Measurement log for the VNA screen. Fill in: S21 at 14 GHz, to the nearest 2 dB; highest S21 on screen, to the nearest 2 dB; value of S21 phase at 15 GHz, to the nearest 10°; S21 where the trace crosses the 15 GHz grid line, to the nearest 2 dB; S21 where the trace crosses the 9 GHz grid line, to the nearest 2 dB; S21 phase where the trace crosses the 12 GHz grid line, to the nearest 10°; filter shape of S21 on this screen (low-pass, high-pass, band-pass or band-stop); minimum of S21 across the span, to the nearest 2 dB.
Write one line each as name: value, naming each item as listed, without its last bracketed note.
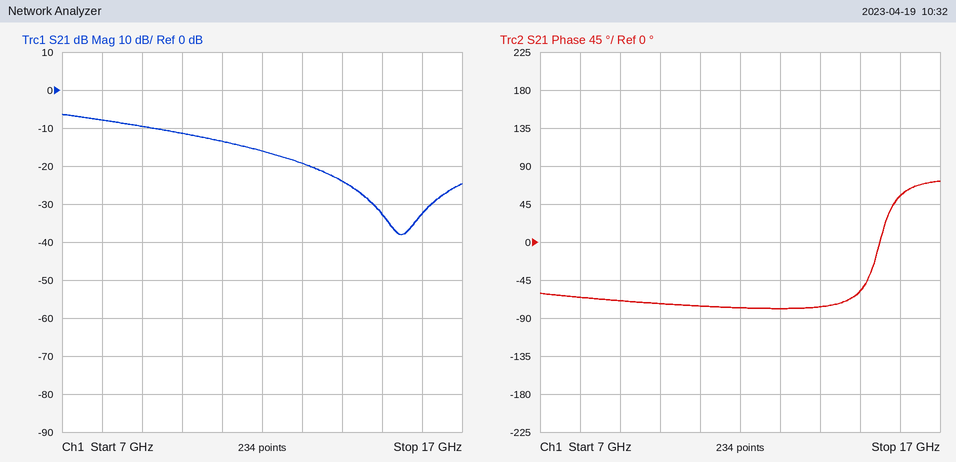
S21 at 14 GHz, to the nearest 2 dB: -24 dB
highest S21 on screen, to the nearest 2 dB: -6 dB
value of S21 phase at 15 GHz, to the nearest 10°: -60°
S21 where the trace crosses the 15 GHz grid line, to the nearest 2 dB: -32 dB
S21 where the trace crosses the 9 GHz grid line, to the nearest 2 dB: -10 dB
S21 phase where the trace crosses the 12 GHz grid line, to the nearest 10°: -80°
filter shape of S21 on this screen: low-pass
minimum of S21 across the span, to the nearest 2 dB: -38 dB
